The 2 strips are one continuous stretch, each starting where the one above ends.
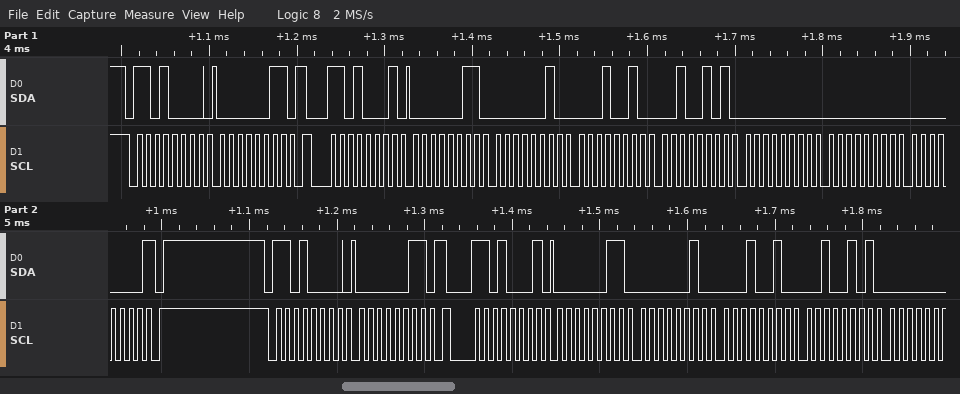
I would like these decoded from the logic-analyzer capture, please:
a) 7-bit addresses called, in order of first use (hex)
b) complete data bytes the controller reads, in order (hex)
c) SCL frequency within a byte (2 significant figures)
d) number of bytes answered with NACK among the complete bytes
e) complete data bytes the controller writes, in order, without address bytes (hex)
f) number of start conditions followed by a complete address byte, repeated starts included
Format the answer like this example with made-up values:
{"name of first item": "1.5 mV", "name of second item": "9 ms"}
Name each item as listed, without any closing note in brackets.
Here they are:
{"7-bit addresses called, in order of first use": "0x68", "complete data bytes the controller reads, in order": "03 02 12 25 00 00 00 03 02 12 25", "SCL frequency within a byte": "100 kHz", "number of bytes answered with NACK among the complete bytes": "1", "complete data bytes the controller writes, in order, without address bytes": "03 03", "number of start conditions followed by a complete address byte, repeated starts included": "4"}
